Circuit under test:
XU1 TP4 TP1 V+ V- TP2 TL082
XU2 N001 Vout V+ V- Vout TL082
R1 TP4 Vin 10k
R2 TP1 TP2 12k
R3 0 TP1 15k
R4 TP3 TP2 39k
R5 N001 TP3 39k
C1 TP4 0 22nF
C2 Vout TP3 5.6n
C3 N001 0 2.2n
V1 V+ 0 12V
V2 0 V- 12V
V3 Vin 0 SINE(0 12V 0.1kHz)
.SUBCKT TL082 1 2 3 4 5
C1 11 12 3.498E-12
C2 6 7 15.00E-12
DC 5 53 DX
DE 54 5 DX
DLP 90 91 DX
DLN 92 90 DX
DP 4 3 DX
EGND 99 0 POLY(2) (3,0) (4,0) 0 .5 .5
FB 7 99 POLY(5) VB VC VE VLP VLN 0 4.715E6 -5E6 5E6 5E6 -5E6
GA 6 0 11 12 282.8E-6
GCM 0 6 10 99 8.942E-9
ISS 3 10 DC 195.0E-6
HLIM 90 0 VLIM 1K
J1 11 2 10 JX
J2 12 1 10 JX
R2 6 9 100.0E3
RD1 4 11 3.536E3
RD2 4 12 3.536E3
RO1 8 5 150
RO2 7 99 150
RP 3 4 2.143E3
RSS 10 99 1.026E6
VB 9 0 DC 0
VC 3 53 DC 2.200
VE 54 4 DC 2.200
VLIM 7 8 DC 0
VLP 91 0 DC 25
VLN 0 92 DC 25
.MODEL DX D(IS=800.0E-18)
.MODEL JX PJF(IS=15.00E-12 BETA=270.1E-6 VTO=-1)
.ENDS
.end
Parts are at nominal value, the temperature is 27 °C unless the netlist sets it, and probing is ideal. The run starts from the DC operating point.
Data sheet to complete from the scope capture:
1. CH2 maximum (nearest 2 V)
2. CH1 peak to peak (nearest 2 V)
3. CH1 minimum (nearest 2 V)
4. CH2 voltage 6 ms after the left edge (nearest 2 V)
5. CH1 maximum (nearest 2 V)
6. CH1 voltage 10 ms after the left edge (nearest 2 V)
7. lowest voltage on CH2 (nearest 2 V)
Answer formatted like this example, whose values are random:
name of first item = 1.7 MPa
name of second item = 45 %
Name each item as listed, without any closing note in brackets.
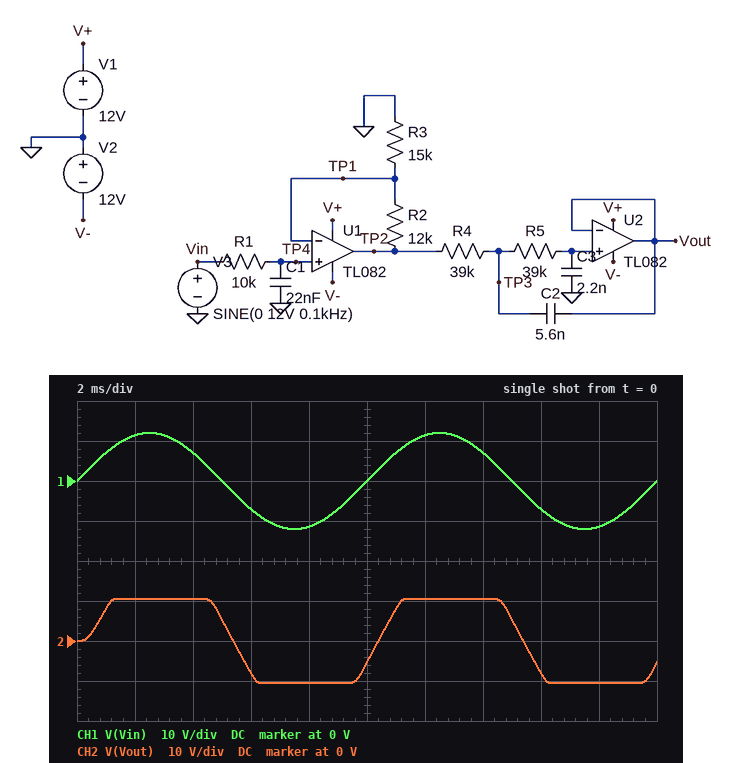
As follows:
CH2 maximum = 10 V
CH1 peak to peak = 24 V
CH1 minimum = -12 V
CH2 voltage 6 ms after the left edge = -8 V
CH1 maximum = 12 V
CH1 voltage 10 ms after the left edge = 0 V
lowest voltage on CH2 = -10 V
